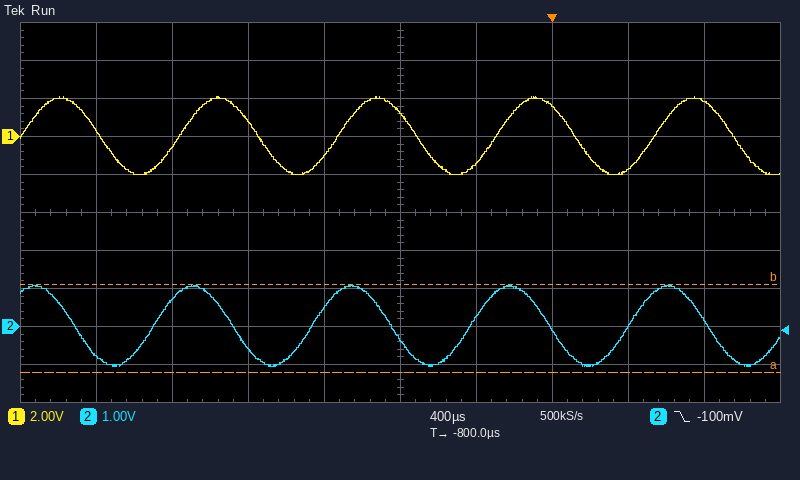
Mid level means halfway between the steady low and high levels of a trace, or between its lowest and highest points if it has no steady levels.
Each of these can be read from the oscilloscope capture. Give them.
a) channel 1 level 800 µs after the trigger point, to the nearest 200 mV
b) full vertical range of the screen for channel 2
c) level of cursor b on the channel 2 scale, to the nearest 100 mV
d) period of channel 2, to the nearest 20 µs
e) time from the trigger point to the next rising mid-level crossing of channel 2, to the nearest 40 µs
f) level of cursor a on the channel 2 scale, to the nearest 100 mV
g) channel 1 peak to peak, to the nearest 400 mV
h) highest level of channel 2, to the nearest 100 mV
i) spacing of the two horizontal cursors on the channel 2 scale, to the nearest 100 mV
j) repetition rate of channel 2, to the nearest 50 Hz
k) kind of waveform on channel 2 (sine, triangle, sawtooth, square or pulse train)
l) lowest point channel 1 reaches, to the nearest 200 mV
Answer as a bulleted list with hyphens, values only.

- 1.8 V
- 10 V
- 1.1 V
- 840 µs
- 400 µs
- -1.2 V
- 4.0 V
- 1.1 V
- 2.3 V
- 1.20 kHz
- sine
- -2.0 V
